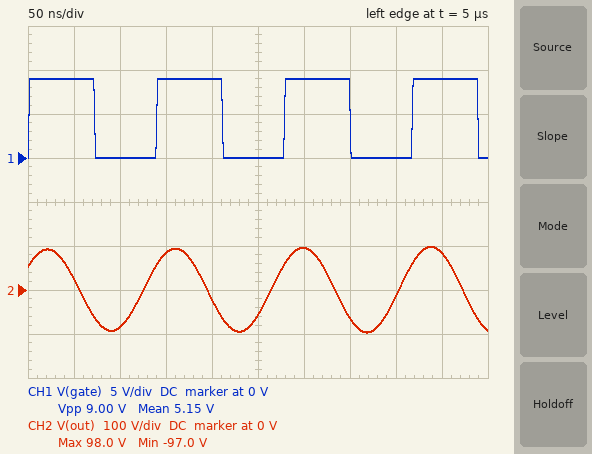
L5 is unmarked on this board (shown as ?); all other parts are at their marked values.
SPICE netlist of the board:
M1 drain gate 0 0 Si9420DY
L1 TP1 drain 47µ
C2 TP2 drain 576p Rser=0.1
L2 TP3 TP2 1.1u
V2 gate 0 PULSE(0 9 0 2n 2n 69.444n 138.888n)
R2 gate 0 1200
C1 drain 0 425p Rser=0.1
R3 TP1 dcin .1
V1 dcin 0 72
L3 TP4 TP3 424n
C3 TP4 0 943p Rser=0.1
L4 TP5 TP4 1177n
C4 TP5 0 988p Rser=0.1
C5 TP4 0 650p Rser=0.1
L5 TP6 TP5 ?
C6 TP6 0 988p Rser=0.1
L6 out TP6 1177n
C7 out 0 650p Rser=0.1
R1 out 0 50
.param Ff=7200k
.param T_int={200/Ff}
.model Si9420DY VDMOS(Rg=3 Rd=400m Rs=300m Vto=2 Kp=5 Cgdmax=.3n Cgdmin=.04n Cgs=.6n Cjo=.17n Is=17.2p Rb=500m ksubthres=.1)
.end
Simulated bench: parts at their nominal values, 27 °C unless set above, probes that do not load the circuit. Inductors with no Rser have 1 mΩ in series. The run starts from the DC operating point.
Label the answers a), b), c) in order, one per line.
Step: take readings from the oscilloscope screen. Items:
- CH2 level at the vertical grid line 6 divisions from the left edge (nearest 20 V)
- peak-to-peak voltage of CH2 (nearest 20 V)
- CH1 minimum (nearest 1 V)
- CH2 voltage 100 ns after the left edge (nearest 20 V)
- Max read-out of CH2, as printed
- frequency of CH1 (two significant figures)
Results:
a) 100 V
b) 200 V
c) 0 V
d) -80 V
e) 98.0 V
f) 7.2 MHz
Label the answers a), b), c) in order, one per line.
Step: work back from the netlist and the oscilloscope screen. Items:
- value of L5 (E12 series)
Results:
a) 2.7 µH
